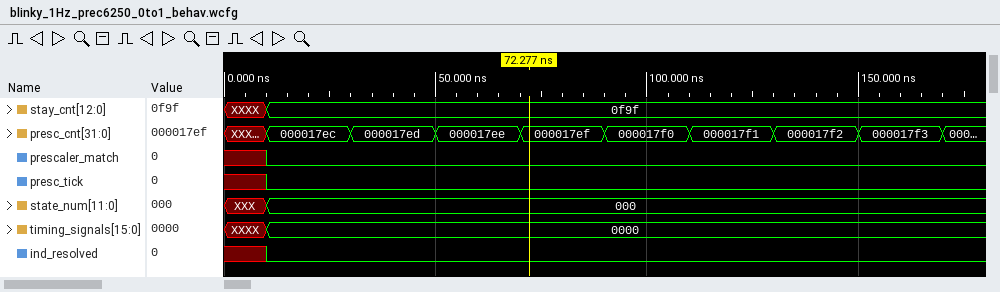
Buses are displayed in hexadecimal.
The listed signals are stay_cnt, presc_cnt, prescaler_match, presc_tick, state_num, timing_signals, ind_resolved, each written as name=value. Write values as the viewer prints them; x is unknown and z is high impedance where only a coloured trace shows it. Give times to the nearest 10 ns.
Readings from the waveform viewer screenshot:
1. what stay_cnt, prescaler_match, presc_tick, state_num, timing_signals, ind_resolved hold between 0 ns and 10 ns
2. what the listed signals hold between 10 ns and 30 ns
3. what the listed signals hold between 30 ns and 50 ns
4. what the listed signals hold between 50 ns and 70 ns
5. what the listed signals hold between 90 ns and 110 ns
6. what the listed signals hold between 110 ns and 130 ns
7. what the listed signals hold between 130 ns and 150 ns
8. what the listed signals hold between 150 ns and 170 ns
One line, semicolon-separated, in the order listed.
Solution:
stay_cnt=XXXX, prescaler_match=x, presc_tick=x, state_num=XXX, timing_signals=XXXX, ind_resolved=x; stay_cnt=0f9f, presc_cnt=000017ec, prescaler_match=0, presc_tick=0, state_num=000, timing_signals=0000, ind_resolved=0; stay_cnt=0f9f, presc_cnt=000017ed, prescaler_match=0, presc_tick=0, state_num=000, timing_signals=0000, ind_resolved=0; stay_cnt=0f9f, presc_cnt=000017ee, prescaler_match=0, presc_tick=0, state_num=000, timing_signals=0000, ind_resolved=0; stay_cnt=0f9f, presc_cnt=000017f0, prescaler_match=0, presc_tick=0, state_num=000, timing_signals=0000, ind_resolved=0; stay_cnt=0f9f, presc_cnt=000017f1, prescaler_match=0, presc_tick=0, state_num=000, timing_signals=0000, ind_resolved=0; stay_cnt=0f9f, presc_cnt=000017f2, prescaler_match=0, presc_tick=0, state_num=000, timing_signals=0000, ind_resolved=0; stay_cnt=0f9f, presc_cnt=000017f3, prescaler_match=0, presc_tick=0, state_num=000, timing_signals=0000, ind_resolved=0
